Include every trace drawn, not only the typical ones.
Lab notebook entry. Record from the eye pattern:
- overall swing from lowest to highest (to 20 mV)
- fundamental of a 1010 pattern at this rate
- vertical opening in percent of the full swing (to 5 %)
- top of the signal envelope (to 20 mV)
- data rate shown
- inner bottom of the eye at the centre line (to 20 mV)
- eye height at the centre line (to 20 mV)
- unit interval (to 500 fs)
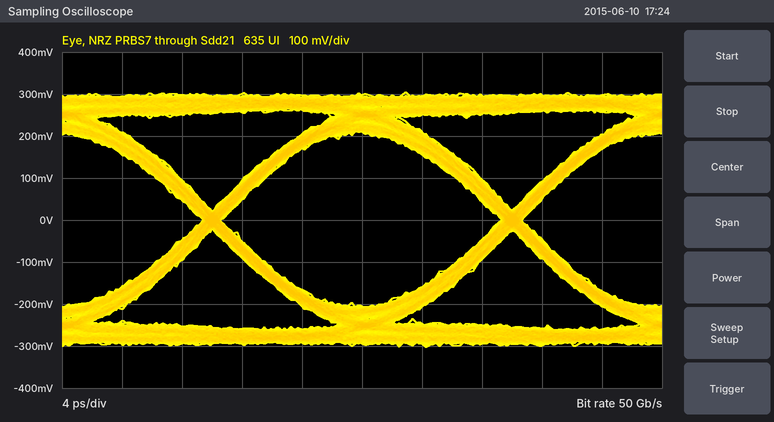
600 mV
25 GHz
70 %
300 mV
50 Gb/s
-200 mV
420 mV
20.0 ps
